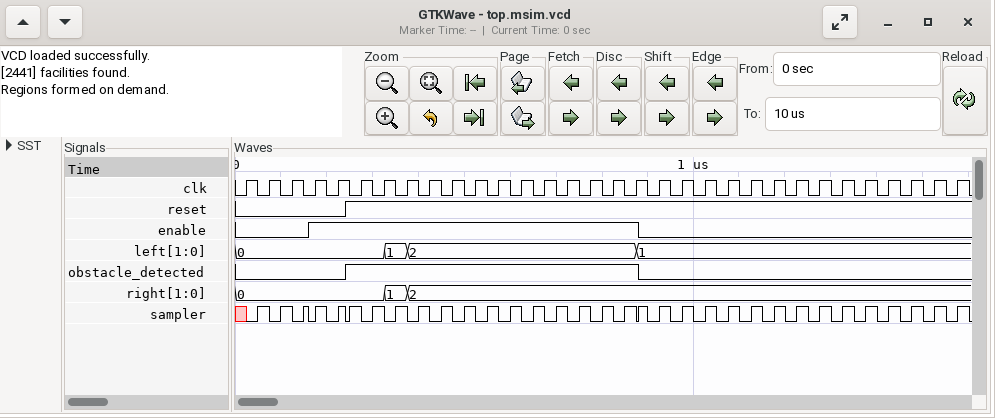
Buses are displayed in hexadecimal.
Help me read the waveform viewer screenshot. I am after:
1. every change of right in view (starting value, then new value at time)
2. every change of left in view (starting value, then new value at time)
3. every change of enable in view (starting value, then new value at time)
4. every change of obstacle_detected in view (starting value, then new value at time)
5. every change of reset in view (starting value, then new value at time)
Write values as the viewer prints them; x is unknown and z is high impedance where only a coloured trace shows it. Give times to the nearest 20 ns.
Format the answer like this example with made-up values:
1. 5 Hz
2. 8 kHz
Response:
1. 0, 1 at 320 ns, 2 at 380 ns
2. 0, 1 at 320 ns, 2 at 380 ns, 1 at 880 ns
3. 0, 1 at 160 ns, 0 at 880 ns
4. 0, 1 at 240 ns, 0 at 880 ns
5. 0, 1 at 240 ns
